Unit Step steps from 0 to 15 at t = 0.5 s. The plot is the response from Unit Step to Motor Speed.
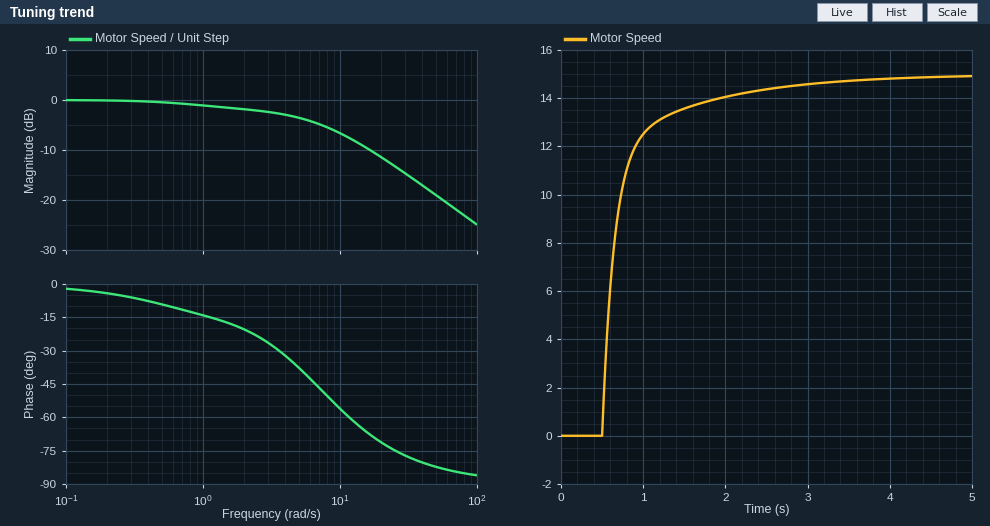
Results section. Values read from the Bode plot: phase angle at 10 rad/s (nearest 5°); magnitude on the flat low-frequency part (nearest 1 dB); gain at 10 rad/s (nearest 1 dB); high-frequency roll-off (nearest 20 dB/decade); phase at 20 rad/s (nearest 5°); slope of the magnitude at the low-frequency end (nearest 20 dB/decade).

-55°
0 dB
-7 dB
-20 dB/decade
-70°
0 dB/decade
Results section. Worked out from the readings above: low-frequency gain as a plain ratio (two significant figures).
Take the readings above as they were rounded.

1.0
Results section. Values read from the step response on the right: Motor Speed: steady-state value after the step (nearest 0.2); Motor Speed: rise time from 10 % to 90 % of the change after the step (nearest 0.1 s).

15.0
0.9 s
